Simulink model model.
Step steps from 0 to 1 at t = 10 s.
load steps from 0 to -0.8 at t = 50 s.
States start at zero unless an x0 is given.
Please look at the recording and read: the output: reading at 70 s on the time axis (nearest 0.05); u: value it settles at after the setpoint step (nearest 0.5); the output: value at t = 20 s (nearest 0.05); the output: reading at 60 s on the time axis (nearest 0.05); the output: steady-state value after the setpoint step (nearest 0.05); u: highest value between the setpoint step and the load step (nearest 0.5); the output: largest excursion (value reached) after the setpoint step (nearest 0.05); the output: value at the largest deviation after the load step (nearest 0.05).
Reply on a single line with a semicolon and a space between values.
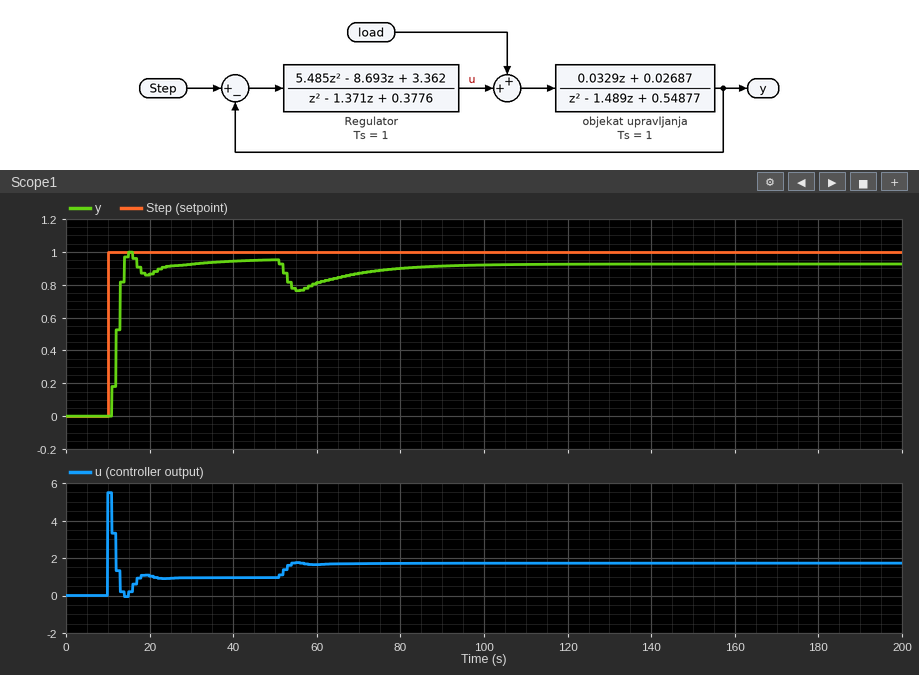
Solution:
0.85; 1.0; 0.85; 0.80; 0.95; 5.5; 1.00; 0.75
